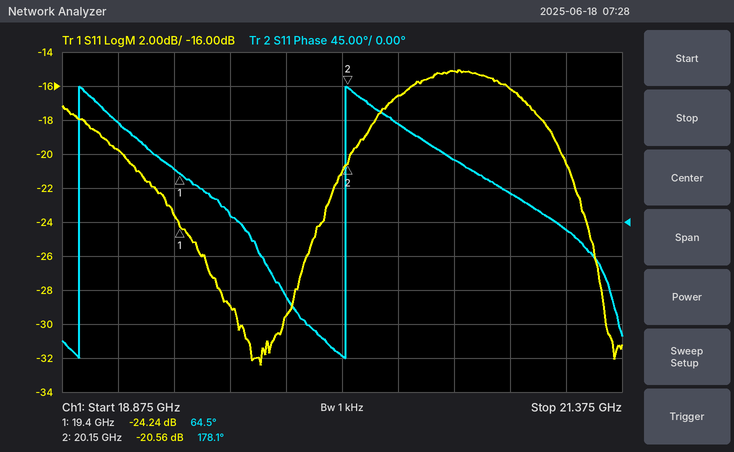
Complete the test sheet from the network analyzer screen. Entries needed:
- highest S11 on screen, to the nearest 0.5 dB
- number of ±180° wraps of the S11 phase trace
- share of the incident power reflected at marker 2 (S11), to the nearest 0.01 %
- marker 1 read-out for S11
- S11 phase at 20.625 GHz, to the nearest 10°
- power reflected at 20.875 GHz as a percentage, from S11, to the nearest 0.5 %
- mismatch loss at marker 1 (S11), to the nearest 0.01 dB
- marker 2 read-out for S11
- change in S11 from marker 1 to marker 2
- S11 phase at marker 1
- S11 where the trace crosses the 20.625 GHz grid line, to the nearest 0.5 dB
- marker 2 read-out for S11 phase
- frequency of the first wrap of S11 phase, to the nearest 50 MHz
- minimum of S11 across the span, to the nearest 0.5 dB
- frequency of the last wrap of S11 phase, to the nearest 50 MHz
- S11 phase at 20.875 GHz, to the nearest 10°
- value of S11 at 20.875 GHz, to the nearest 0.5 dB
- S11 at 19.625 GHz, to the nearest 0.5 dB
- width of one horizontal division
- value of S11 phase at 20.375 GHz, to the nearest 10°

-15.0 dB
2
0.88 %
-24.24 dB
80°
2.5 %
0.02 dB
-20.56 dB
3.68 dB
64.5°
-15.0 dB
178.1°
18.95 GHz
-32.5 dB
20.15 GHz
40°
-16.0 dB
-29.0 dB
250 MHz
130°
